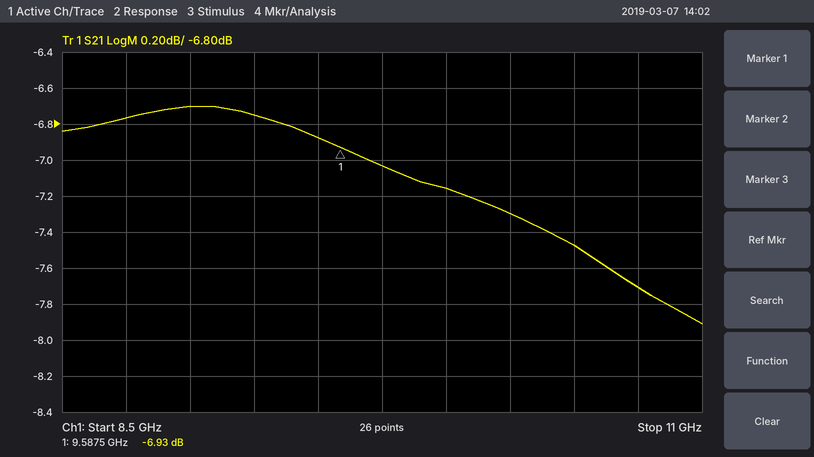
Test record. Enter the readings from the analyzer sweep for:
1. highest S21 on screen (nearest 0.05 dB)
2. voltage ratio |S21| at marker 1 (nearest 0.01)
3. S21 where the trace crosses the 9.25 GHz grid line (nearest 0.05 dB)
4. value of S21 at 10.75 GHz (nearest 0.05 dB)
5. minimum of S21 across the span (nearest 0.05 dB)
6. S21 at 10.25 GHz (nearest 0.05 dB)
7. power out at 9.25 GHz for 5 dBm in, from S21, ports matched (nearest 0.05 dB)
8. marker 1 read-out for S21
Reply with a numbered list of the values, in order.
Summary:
1. -6.70 dB
2. 0.45
3. -6.75 dB
4. -7.70 dB
5. -7.90 dB
6. -7.30 dB
7. -1.75 dBm
8. -6.93 dB
